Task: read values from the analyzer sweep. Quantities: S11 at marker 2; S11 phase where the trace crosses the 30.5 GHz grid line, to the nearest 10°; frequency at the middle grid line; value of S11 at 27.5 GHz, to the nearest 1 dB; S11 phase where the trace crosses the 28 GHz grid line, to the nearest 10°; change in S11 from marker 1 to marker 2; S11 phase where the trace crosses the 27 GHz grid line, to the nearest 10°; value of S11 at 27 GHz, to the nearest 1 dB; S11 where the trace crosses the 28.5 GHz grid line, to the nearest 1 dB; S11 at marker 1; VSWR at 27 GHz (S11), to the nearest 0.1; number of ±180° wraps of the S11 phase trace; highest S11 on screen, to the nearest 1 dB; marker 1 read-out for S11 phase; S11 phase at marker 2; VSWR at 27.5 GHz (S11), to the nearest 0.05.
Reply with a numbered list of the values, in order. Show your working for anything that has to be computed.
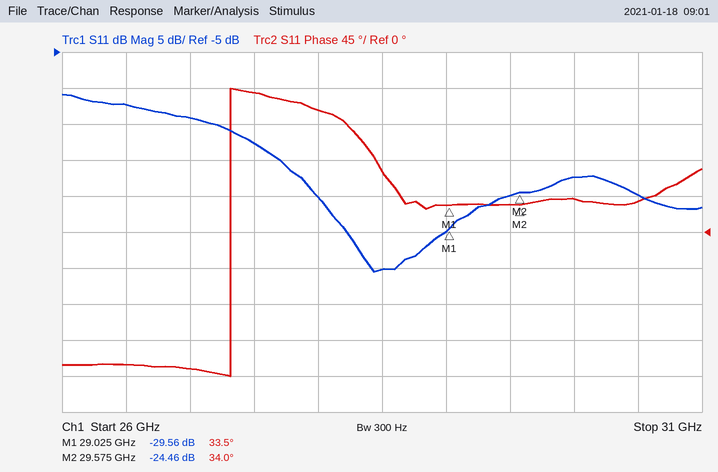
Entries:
1. -24.46 dB
2. 40°
3. 28.5 GHz
4. -18 dB
5. 150°
6. -24.46 − (-29.56) = 5.10 dB
7. -170°
8. -14 dB
9. -35 dB
10. -29.56 dB
11. |Γ| = 10^(-14/20) = 0.1995; VSWR = (1 + 0.1995)/(1 − 0.1995) ≈ 1.5
12. 1
13. -11 dB
14. 33.5°
15. 34.0°
16. |Γ| = 10^(-18/20) = 0.1259; VSWR = (1 + 0.1259)/(1 − 0.1259) ≈ 1.29, so 1.30 to the nearest 0.05
